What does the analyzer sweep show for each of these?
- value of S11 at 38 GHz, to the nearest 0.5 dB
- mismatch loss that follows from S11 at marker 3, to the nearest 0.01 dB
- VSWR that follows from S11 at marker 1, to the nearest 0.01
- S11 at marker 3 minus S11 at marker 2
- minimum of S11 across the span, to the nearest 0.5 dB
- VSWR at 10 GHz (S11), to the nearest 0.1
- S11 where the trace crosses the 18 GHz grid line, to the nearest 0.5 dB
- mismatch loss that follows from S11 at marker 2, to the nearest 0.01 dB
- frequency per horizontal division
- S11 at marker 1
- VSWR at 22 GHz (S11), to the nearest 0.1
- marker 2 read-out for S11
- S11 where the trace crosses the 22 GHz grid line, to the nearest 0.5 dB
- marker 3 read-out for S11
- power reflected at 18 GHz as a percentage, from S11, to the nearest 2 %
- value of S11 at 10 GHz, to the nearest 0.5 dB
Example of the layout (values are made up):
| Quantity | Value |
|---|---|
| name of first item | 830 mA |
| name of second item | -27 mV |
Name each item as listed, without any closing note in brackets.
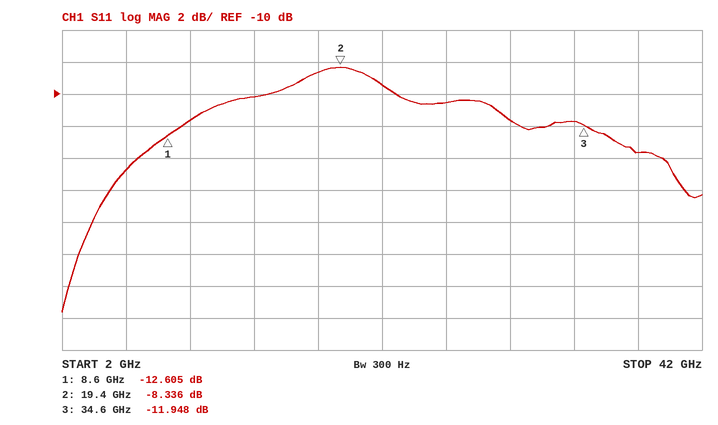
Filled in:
| Quantity | Value |
|---|---|
| value of S11 at 38 GHz, to the nearest 0.5 dB | -13.5 dB |
| mismatch loss that follows from S11 at marker 3, to the nearest 0.01 dB | 0.29 dB |
| VSWR that follows from S11 at marker 1, to the nearest 0.01 | 1.61 |
| S11 at marker 3 minus S11 at marker 2 | -3.612 dB |
| minimum of S11 across the span, to the nearest 0.5 dB | -23.5 dB |
| VSWR at 10 GHz (S11), to the nearest 0.1 | 1.7 |
| S11 where the trace crosses the 18 GHz grid line, to the nearest 0.5 dB | -8.5 dB |
| mismatch loss that follows from S11 at marker 2, to the nearest 0.01 dB | 0.69 dB |
| frequency per horizontal division | 4 GHz |
| S11 at marker 1 | -12.605 dB |
| VSWR at 22 GHz (S11), to the nearest 0.1 | 2.0 |
| marker 2 read-out for S11 | -8.336 dB |
| S11 where the trace crosses the 22 GHz grid line, to the nearest 0.5 dB | -9.5 dB |
| marker 3 read-out for S11 | -11.948 dB |
| power reflected at 18 GHz as a percentage, from S11, to the nearest 2 % | 14 % |
| value of S11 at 10 GHz, to the nearest 0.5 dB | -11.5 dB |
